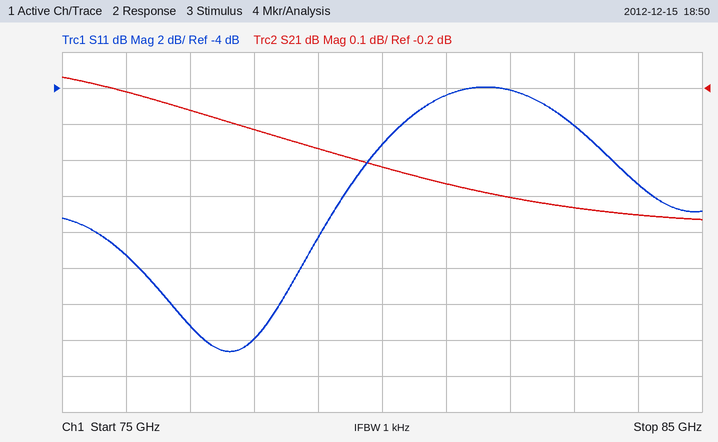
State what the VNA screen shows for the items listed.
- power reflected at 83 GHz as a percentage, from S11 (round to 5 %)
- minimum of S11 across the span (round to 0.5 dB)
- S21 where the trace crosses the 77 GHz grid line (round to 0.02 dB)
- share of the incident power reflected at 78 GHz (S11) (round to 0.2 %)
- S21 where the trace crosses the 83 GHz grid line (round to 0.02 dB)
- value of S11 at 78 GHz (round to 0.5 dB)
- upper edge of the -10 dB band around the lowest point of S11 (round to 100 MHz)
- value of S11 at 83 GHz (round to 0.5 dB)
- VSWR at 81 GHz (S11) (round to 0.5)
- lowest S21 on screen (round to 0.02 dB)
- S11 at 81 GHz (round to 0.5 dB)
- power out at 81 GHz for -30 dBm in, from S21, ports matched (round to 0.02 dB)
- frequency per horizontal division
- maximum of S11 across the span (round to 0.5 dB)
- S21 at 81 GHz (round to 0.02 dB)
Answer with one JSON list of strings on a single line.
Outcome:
["25 %", "-18.5 dB", "-0.26 dB", "1.6 %", "-0.54 dB", "-18.0 dB", "79.4 GHz", "-6.0 dB", "4.0", "-0.56 dB", "-4.5 dB", "-30.46 dBm", "1 GHz", "-4.0 dB", "-0.46 dB"]
